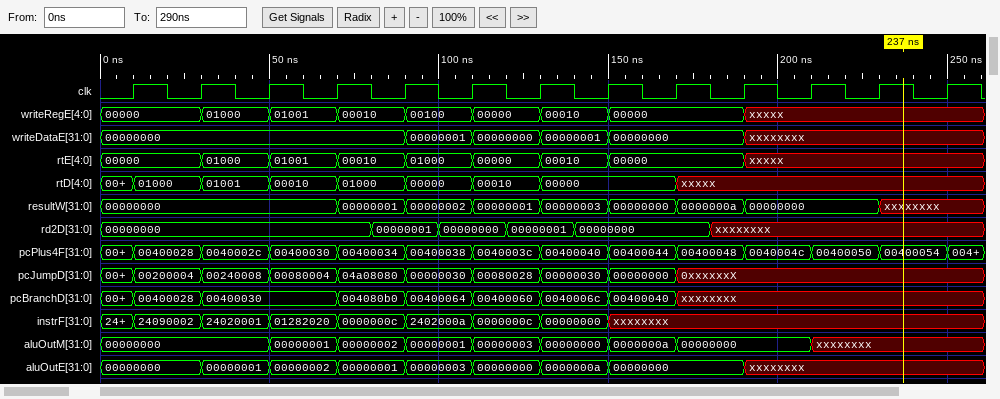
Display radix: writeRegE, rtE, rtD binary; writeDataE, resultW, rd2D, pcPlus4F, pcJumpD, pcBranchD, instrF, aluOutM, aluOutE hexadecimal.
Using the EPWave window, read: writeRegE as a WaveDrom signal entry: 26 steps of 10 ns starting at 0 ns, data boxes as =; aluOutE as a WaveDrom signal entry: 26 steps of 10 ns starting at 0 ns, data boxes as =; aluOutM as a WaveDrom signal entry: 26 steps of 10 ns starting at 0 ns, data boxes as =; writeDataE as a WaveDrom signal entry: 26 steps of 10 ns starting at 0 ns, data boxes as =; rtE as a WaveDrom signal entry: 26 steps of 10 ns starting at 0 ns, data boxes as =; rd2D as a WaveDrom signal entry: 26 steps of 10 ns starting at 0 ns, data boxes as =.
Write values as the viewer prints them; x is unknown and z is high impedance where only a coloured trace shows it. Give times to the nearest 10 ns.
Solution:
{name: 'writeRegE', wave: '=..=.=.=.=.=.=.=...x......', data: '00000 01000 01001 00010 00100 00000 00010 00000'}
{name: 'aluOutE', wave: '=..=.=.=.=.=.=.=...x......', data: '00000000 00000001 00000002 00000001 00000003 00000000 0000000a 00000000'}
{name: 'aluOutM', wave: '=....=.=.=.=.=.=.=...x....', data: '00000000 00000001 00000002 00000001 00000003 00000000 0000000a 00000000'}
{name: 'writeDataE', wave: '=........=.=.=.=...x......', data: '00000000 00000001 00000000 00000001 00000000'}
{name: 'rtE', wave: '=..=.=.=.=.=.=.=...x......', data: '00000 01000 01001 00010 01000 00000 00010 00000'}
{name: 'rd2D', wave: '=.......=.=.=.=...x.......', data: '00000000 00000001 00000000 00000001 00000000'}
